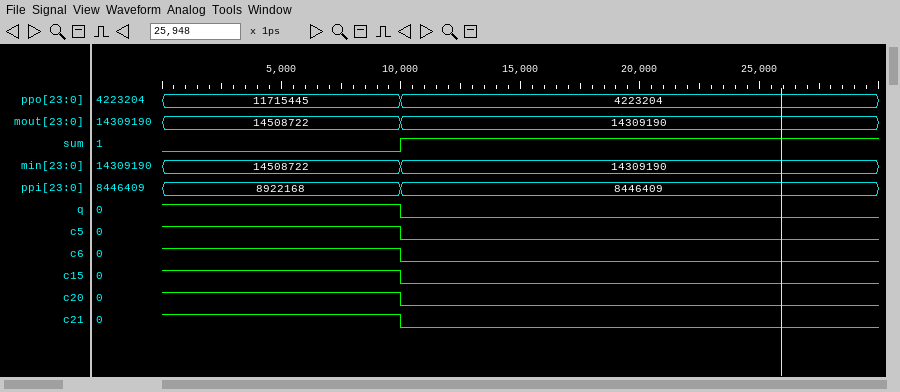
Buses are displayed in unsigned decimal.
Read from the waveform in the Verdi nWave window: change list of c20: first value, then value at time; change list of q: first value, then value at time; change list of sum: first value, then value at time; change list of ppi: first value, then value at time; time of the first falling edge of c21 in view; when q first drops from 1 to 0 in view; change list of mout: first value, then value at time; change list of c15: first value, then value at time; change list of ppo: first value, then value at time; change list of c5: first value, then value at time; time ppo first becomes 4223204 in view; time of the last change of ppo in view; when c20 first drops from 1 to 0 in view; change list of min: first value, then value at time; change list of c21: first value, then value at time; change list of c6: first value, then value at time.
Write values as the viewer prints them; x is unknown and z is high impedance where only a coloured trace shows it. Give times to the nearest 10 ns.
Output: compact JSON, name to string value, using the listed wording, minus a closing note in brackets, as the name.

{"change list of c20: first value, then value at time": "1, 0 at 10 ns", "change list of q: first value, then value at time": "1, 0 at 10 ns", "change list of sum: first value, then value at time": "0, 1 at 10 ns", "change list of ppi: first value, then value at time": "8922168, 8446409 at 10 ns", "time of the first falling edge of c21 in view": "10 ns", "when q first drops from 1 to 0 in view": "10 ns", "change list of mout: first value, then value at time": "14508722, 14309190 at 10 ns", "change list of c15: first value, then value at time": "1, 0 at 10 ns", "change list of ppo: first value, then value at time": "11715445, 4223204 at 10 ns", "change list of c5: first value, then value at time": "1, 0 at 10 ns", "time ppo first becomes 4223204 in view": "10 ns", "time of the last change of ppo in view": "10 ns", "when c20 first drops from 1 to 0 in view": "10 ns", "change list of min: first value, then value at time": "14508722, 14309190 at 10 ns", "change list of c21: first value, then value at time": "1, 0 at 10 ns", "change list of c6: first value, then value at time": "1, 0 at 10 ns"}
